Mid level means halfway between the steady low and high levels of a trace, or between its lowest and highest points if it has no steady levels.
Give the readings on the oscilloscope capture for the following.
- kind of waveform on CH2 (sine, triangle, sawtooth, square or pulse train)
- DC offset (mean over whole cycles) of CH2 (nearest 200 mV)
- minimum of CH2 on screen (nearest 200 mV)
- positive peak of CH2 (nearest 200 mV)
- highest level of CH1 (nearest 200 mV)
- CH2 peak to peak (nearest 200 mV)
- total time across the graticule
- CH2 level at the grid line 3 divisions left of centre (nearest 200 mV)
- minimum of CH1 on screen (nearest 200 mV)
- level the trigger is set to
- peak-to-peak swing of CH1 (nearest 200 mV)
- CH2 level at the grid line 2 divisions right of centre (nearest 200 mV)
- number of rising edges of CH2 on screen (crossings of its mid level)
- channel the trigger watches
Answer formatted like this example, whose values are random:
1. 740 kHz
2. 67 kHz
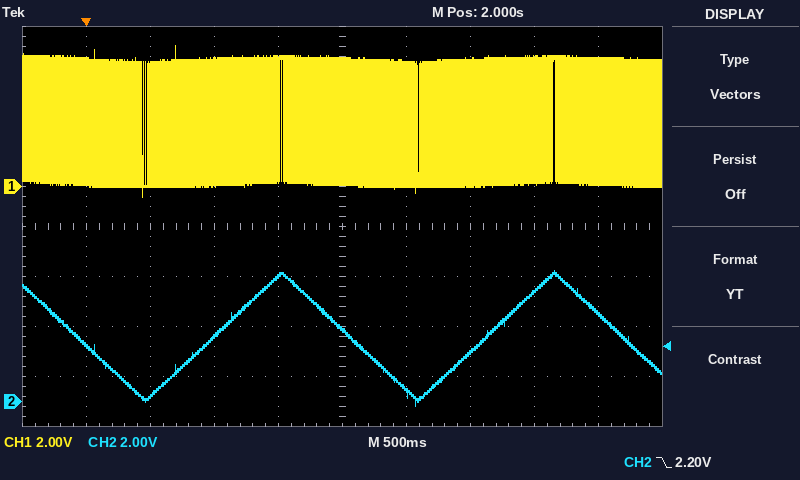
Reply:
1. triangle
2. 2.6 V
3. -200 mV
4. 5.2 V
5. 5.6 V
6. 5.4 V
7. 5 s
8. 200 mV
9. -400 mV
10. 2.20 V
11. 6.0 V
12. 2.0 V
13. 2
14. CH2
